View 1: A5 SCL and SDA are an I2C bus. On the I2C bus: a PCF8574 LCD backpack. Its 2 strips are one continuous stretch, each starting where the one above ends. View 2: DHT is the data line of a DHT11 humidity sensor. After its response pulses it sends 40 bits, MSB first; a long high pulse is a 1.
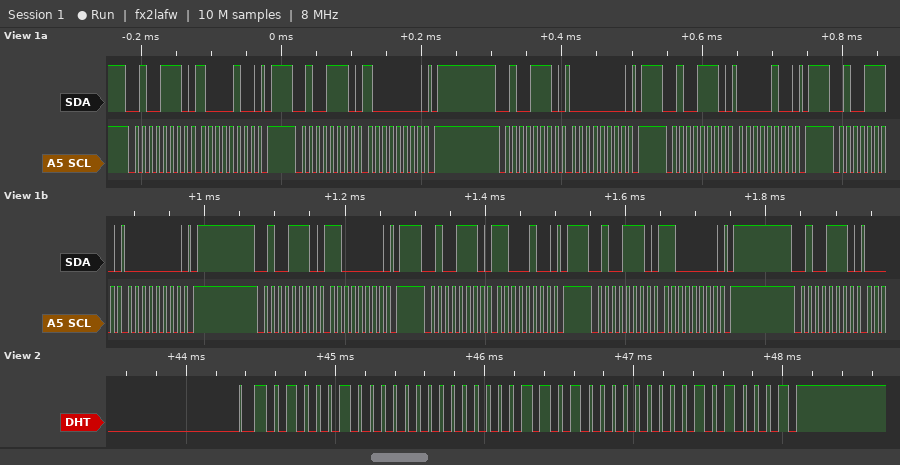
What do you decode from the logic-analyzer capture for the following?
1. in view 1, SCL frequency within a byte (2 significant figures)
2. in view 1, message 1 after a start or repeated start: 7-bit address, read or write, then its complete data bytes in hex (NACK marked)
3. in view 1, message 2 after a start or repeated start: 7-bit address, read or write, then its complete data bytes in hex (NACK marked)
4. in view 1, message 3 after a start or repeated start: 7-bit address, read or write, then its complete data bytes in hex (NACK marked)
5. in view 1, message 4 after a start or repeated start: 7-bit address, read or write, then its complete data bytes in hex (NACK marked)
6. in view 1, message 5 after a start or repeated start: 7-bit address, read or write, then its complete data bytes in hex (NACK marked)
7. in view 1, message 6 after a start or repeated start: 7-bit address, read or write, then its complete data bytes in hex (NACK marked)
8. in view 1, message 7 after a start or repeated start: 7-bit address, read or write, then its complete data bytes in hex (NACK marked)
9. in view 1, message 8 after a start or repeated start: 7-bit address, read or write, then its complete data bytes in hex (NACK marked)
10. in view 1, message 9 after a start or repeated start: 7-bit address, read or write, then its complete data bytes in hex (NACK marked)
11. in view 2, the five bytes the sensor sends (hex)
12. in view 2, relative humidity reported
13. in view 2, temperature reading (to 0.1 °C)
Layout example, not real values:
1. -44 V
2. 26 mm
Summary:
1. 100 kHz
2. 0x27 write: 84
3. 0x27 write: 80
4. 0x27 write: 00
5. 0x27 write: 04
6. 0x27 write: 00
7. 0x27 write: C0
8. 0x27 write: C4
9. 0x27 write: C0
10. 0x27 write
11. 44 00 0D 00 51
12. 68 %
13. 13.0 °C
